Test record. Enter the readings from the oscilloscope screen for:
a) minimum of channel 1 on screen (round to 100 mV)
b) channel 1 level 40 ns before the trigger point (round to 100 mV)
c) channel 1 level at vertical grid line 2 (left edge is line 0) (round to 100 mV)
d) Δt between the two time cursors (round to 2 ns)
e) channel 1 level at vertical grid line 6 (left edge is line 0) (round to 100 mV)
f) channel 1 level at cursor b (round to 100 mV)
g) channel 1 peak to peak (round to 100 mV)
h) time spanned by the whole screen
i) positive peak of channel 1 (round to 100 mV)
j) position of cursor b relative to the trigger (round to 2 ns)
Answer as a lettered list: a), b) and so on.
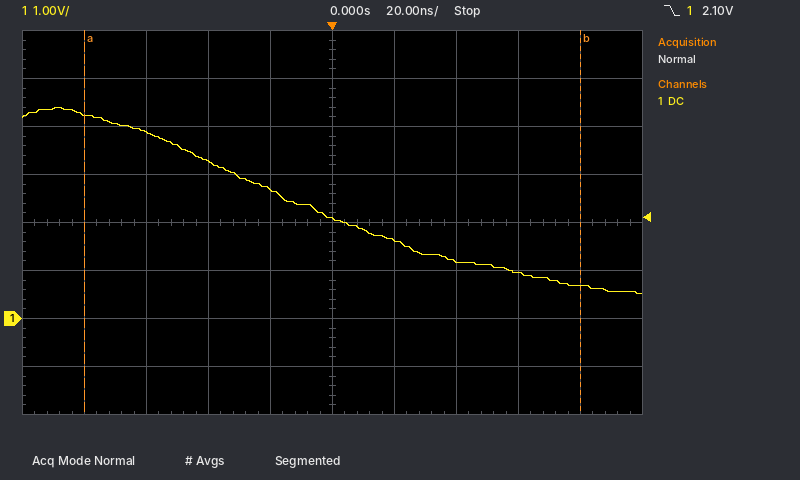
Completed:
a) 500 mV
b) 3.3 V
c) 3.9 V
d) 160 ns
e) 1.6 V
f) 700 mV
g) 3.9 V
h) 200 ns
i) 4.4 V
j) +80 ns
